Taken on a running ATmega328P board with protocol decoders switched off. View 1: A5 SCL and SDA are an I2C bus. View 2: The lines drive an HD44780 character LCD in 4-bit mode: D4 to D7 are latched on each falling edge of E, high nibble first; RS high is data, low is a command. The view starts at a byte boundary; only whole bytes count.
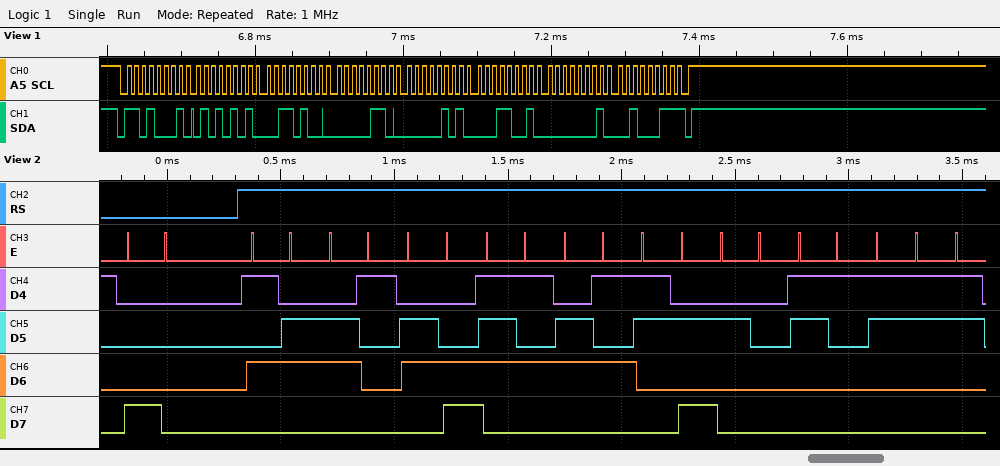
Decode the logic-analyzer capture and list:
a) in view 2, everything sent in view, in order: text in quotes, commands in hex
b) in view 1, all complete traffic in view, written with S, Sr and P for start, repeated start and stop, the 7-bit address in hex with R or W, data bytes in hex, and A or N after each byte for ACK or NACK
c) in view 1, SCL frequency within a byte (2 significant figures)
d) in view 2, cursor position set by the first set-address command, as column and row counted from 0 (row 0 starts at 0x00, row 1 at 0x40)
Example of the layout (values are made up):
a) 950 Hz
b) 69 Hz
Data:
a) 0x80 "Value: 13"
b) S 68R A 55 A 34 A 06 A 05 A 19 A 01 A 23 N P
c) 100 kHz
d) column 0, row 0
